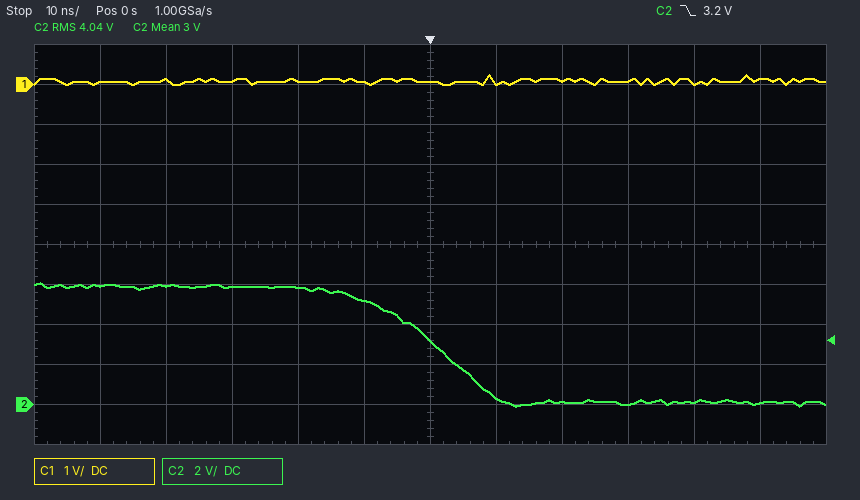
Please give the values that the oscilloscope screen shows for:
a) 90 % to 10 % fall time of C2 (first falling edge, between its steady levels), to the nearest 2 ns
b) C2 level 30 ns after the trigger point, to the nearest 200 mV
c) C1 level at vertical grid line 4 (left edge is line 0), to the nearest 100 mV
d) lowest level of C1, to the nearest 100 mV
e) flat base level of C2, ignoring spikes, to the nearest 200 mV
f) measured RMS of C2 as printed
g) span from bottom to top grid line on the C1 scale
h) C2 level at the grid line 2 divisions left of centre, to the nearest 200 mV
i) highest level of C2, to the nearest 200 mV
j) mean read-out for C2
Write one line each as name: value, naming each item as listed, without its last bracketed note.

90 % to 10 % fall time of C2 (first falling edge, between its steady levels), to the nearest 2 ns: 20 ns
C2 level 30 ns after the trigger point, to the nearest 200 mV: 0.0 V
C1 level at vertical grid line 4 (left edge is line 0), to the nearest 100 mV: 100 mV
lowest level of C1, to the nearest 100 mV: 0.0 V
flat base level of C2, ignoring spikes, to the nearest 200 mV: 200 mV
measured RMS of C2 as printed: 4.04 V
span from bottom to top grid line on the C1 scale: 10 V
C2 level at the grid line 2 divisions left of centre, to the nearest 200 mV: 5.8 V
highest level of C2, to the nearest 200 mV: 6.0 V
mean read-out for C2: 3 V
